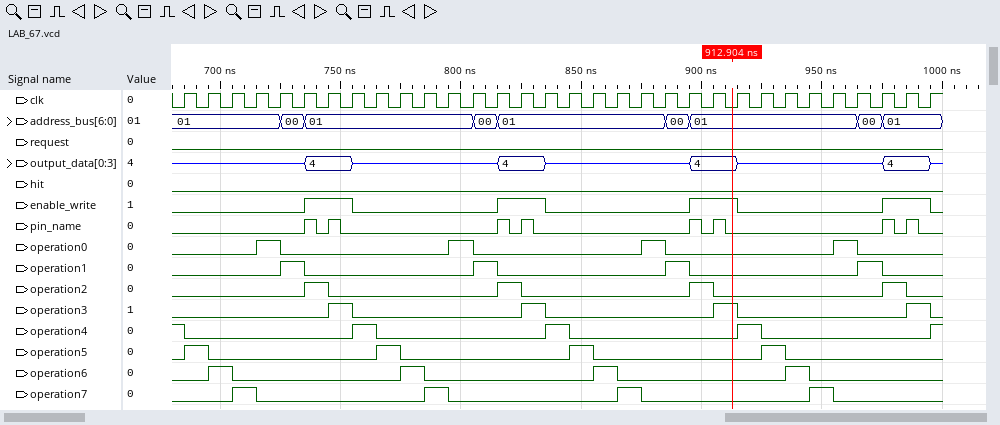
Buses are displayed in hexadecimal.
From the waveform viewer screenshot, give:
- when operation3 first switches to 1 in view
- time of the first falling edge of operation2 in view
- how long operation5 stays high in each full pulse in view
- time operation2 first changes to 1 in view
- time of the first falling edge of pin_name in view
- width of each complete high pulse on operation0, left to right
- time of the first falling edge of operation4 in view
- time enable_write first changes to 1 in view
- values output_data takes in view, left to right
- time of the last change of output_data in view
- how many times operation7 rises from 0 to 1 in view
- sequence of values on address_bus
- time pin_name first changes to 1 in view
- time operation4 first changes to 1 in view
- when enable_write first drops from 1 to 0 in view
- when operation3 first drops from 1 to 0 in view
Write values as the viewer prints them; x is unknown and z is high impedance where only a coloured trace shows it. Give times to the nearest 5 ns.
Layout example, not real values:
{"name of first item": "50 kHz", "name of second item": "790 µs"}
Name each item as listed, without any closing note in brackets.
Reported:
{"when operation3 first switches to 1 in view": "745 ns", "time of the first falling edge of operation2 in view": "745 ns", "how long operation5 stays high in each full pulse in view": "10 ns, 10 ns, 10 ns, 10 ns", "time operation2 first changes to 1 in view": "735 ns", "time of the first falling edge of pin_name in view": "740 ns", "width of each complete high pulse on operation0, left to right": "10 ns, 10 ns, 10 ns, 10 ns", "time of the first falling edge of operation4 in view": "685 ns", "time enable_write first changes to 1 in view": "735 ns", "values output_data takes in view, left to right": "z, 4, z, 4, z, 4, z, 4, z", "time of the last change of output_data in view": "995 ns", "how many times operation7 rises from 0 to 1 in view": "4", "sequence of values on address_bus": "01, 00, 01, 00, 01, 00, 01, 00, 01", "time pin_name first changes to 1 in view": "735 ns", "time operation4 first changes to 1 in view": "755 ns", "when enable_write first drops from 1 to 0 in view": "755 ns", "when operation3 first drops from 1 to 0 in view": "755 ns"}
